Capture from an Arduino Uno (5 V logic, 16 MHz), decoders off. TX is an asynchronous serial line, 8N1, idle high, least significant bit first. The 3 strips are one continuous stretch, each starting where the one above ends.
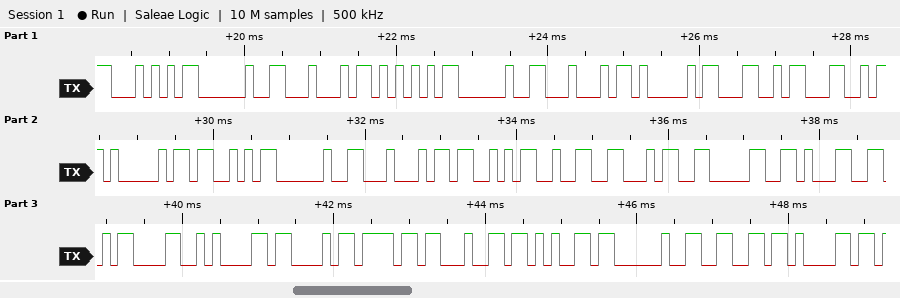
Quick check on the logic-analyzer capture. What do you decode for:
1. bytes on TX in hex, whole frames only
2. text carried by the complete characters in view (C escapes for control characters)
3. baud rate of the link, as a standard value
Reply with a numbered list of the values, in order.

1. 54 20 44 55 20 44 41 4C 4C 41 53 20 44 53 32 34 30 31 0D 0A 43 6F 64 65 20 66 61
2. "T DU DALLAS DS2401\r\nCode fa"
3. 9600 baud
